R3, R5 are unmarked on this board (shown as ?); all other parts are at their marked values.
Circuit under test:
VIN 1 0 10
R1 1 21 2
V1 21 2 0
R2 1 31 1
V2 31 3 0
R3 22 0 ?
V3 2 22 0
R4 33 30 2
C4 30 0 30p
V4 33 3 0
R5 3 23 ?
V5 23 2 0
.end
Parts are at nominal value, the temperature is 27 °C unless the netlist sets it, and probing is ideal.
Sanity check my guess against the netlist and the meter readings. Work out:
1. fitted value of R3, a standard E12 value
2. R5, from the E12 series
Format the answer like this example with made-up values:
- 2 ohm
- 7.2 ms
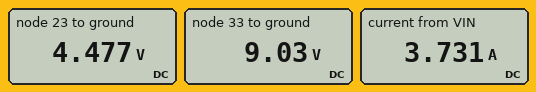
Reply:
- 1.2 Ω
- 4.7 Ω
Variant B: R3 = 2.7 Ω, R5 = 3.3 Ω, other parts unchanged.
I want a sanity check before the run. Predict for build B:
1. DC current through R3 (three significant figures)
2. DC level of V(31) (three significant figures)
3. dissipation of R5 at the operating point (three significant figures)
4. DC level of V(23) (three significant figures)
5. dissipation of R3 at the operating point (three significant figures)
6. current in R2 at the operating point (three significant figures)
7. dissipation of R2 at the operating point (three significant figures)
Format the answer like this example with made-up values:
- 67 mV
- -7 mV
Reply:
- 2.46 A
- 9.22 V
- 2.01 W
- 6.64 V
- 16.3 W
- 781 mA
- 610 mW
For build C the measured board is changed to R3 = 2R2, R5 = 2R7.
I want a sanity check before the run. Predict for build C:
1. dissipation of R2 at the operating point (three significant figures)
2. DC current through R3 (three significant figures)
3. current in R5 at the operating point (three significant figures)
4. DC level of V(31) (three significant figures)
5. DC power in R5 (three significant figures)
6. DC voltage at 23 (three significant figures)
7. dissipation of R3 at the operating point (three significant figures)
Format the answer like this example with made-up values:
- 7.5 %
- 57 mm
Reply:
- 1.01 W
- 2.86 A
- 1.00 A
- 9.00 V
- 2.72 W
- 6.29 V
- 18.0 W
